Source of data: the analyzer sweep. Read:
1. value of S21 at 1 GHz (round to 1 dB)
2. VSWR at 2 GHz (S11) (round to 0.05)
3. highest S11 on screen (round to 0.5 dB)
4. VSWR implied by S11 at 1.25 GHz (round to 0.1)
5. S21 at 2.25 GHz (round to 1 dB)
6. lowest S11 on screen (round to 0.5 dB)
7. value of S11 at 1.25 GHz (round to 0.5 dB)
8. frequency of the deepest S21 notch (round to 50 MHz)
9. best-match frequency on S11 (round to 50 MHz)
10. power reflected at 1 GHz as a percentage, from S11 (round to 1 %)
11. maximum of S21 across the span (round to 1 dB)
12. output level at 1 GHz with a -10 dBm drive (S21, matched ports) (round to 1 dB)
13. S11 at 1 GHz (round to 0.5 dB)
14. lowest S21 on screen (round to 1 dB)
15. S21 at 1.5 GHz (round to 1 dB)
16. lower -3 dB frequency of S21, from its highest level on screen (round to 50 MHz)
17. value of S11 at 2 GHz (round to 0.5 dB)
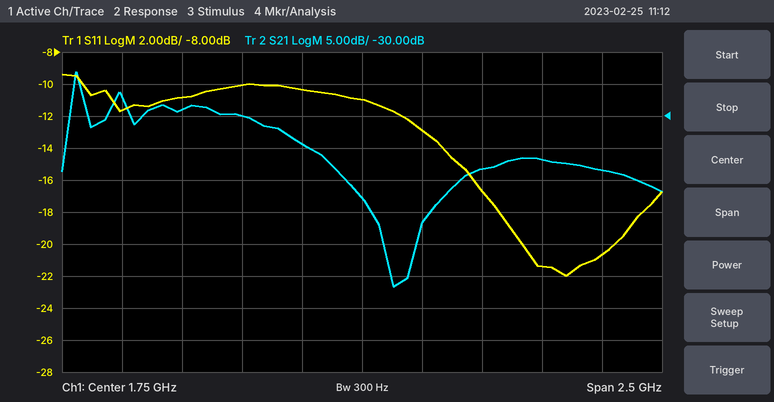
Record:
-29 dB
1.60
-9.5 dB
1.9
-38 dB
-22.0 dB
-10.0 dB
1.90 GHz
2.60 GHz
8 %
-23 dB
-39 dBm
-11.0 dB
-57 dB
-34 dB
550 MHz
-13.0 dB
